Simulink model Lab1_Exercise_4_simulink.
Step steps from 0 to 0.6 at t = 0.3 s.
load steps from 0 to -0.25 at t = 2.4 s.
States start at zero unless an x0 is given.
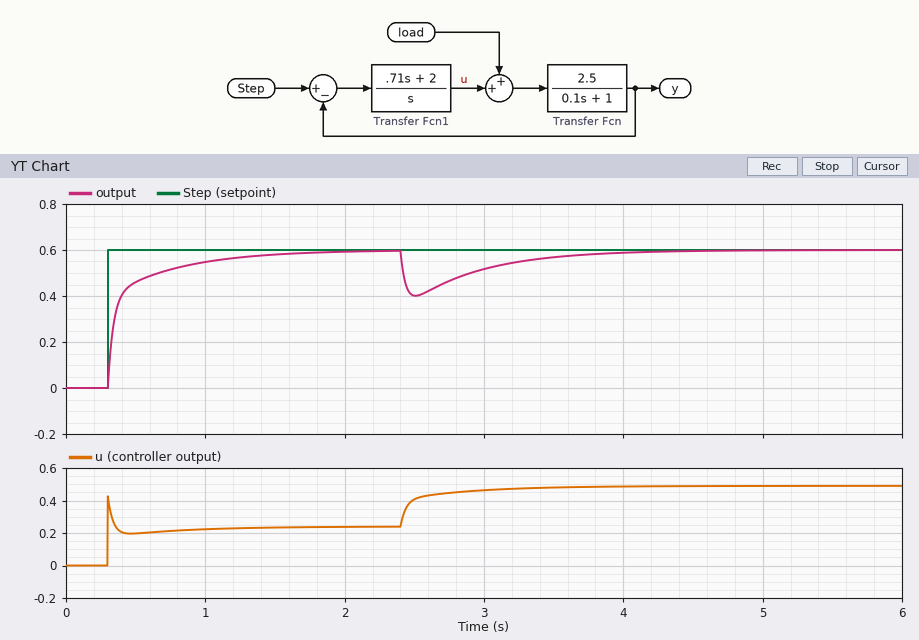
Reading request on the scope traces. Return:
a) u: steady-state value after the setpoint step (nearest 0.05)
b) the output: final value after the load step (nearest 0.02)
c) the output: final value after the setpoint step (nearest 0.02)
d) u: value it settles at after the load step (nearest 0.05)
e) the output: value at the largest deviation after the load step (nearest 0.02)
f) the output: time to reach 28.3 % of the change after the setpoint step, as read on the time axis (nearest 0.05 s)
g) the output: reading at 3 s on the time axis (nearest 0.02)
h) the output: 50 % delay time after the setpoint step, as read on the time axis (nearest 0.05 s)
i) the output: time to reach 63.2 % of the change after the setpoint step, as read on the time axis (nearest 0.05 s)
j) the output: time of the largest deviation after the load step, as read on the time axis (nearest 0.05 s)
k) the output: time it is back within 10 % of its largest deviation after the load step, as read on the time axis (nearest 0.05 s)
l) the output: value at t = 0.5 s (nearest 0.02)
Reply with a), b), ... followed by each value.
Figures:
a) 0.25
b) 0.60
c) 0.60
d) 0.50
e) 0.40
f) 0.30 s
g) 0.52
h) 0.35 s
i) 0.40 s
j) 2.50 s
k) 3.75 s
l) 0.46
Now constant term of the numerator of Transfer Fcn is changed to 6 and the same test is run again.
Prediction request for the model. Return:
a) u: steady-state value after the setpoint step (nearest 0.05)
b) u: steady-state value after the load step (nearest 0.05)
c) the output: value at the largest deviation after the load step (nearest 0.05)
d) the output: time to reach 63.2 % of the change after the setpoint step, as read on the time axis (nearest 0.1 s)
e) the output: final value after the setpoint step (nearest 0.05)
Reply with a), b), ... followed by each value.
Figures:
a) 0.10
b) 0.35
c) 0.35
d) 0.3 s
e) 0.60
